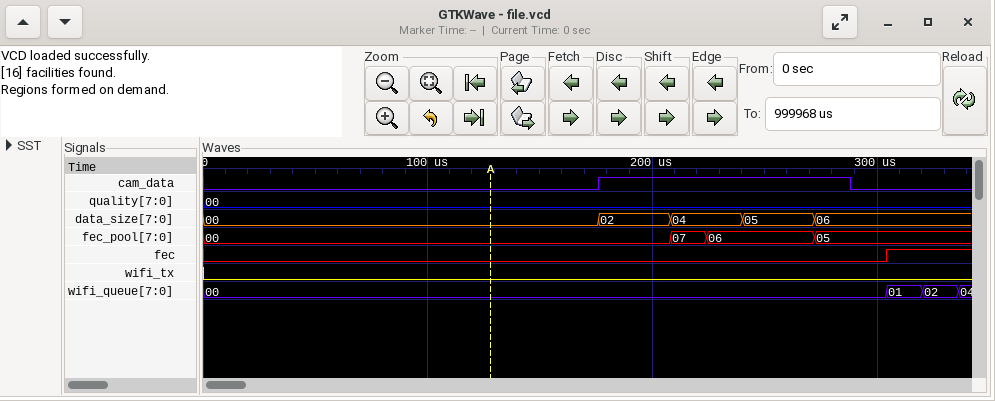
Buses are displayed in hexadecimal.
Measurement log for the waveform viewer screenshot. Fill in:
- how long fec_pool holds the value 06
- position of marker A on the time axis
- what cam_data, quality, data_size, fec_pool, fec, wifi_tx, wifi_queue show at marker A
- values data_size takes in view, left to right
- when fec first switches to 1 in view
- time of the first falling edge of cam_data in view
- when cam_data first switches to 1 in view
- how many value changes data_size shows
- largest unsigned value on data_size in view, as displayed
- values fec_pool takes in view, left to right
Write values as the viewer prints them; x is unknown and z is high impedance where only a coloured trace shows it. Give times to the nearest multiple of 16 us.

48 us
128 us
cam_data=0, quality=00, data_size=00, fec_pool=00, fec=0, wifi_tx=0, wifi_queue=00
00, 02, 04, 05, 06
304 us
288 us
176 us
4
06
00, 07, 06, 05
